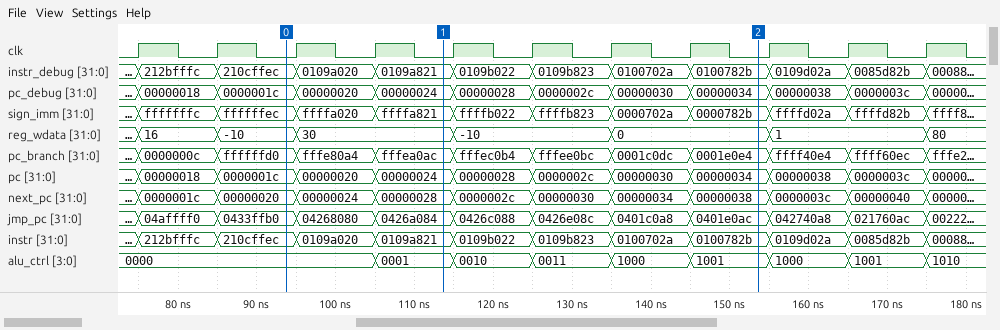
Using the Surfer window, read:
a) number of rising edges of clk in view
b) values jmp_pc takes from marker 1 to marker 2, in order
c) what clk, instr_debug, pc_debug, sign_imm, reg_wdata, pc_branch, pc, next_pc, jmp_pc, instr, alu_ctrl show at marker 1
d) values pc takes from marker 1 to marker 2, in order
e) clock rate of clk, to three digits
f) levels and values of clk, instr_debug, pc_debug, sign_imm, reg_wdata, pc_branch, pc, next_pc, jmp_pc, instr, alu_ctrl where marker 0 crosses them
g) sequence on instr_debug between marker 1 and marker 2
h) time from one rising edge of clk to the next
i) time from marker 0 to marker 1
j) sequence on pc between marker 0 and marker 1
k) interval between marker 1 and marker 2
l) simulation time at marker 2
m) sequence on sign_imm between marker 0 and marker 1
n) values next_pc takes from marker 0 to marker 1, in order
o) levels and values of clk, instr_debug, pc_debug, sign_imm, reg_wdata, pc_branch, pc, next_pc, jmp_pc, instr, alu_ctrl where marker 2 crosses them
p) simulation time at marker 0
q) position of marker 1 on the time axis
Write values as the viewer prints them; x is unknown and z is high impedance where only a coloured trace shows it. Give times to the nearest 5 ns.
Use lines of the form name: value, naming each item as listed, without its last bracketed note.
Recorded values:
number of rising edges of clk in view: 11
values jmp_pc takes from marker 1 to marker 2, in order: 0426a084, 0426c088, 0426e08c, 0401c0a8, 0401e0ac
what clk, instr_debug, pc_debug, sign_imm, reg_wdata, pc_branch, pc, next_pc, jmp_pc, instr, alu_ctrl show at marker 1: clk=0, instr_debug=0109a821, pc_debug=00000024, sign_imm=ffffa821, reg_wdata=30, pc_branch=fffea0ac, pc=00000024, next_pc=00000028, jmp_pc=0426a084, instr=0109a821, alu_ctrl=0001
values pc takes from marker 1 to marker 2, in order: 00000024, 00000028, 0000002c, 00000030, 00000034
clock rate of clk, to three digits: 100 MHz
levels and values of clk, instr_debug, pc_debug, sign_imm, reg_wdata, pc_branch, pc, next_pc, jmp_pc, instr, alu_ctrl where marker 0 crosses them: clk=0, instr_debug=210cffec, pc_debug=0000001c, sign_imm=ffffffec, reg_wdata=-10, pc_branch=ffffffd0, pc=0000001c, next_pc=00000020, jmp_pc=0433ffb0, instr=210cffec, alu_ctrl=0000
sequence on instr_debug between marker 1 and marker 2: 0109a821, 0109b022, 0109b823, 0100702a, 0100782b
time from one rising edge of clk to the next: 10 ns
time from marker 0 to marker 1: 20 ns
sequence on pc between marker 0 and marker 1: 0000001c, 00000020, 00000024
interval between marker 1 and marker 2: 40 ns
simulation time at marker 2: 155 ns
sequence on sign_imm between marker 0 and marker 1: ffffffec, ffffa020, ffffa821
values next_pc takes from marker 0 to marker 1, in order: 00000020, 00000024, 00000028
levels and values of clk, instr_debug, pc_debug, sign_imm, reg_wdata, pc_branch, pc, next_pc, jmp_pc, instr, alu_ctrl where marker 2 crosses them: clk=0, instr_debug=0100782b, pc_debug=00000034, sign_imm=0000782b, reg_wdata=0, pc_branch=0001e0e4, pc=00000034, next_pc=00000038, jmp_pc=0401e0ac, instr=0100782b, alu_ctrl=1001
simulation time at marker 0: 95 ns
position of marker 1 on the time axis: 115 ns
